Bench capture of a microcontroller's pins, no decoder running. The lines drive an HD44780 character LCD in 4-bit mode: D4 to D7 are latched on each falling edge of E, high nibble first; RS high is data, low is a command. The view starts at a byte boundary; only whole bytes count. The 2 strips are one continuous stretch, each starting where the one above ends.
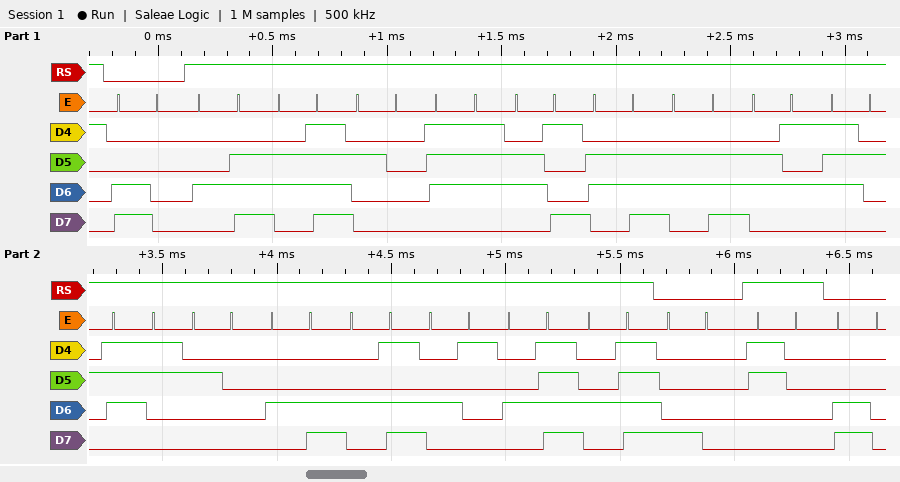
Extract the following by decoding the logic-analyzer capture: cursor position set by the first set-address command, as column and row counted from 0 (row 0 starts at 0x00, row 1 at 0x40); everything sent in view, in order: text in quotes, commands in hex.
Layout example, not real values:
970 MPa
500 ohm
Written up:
column 0, row 1
0xC0 "No winners LMAOO" 0x80 "0" 0xC0
